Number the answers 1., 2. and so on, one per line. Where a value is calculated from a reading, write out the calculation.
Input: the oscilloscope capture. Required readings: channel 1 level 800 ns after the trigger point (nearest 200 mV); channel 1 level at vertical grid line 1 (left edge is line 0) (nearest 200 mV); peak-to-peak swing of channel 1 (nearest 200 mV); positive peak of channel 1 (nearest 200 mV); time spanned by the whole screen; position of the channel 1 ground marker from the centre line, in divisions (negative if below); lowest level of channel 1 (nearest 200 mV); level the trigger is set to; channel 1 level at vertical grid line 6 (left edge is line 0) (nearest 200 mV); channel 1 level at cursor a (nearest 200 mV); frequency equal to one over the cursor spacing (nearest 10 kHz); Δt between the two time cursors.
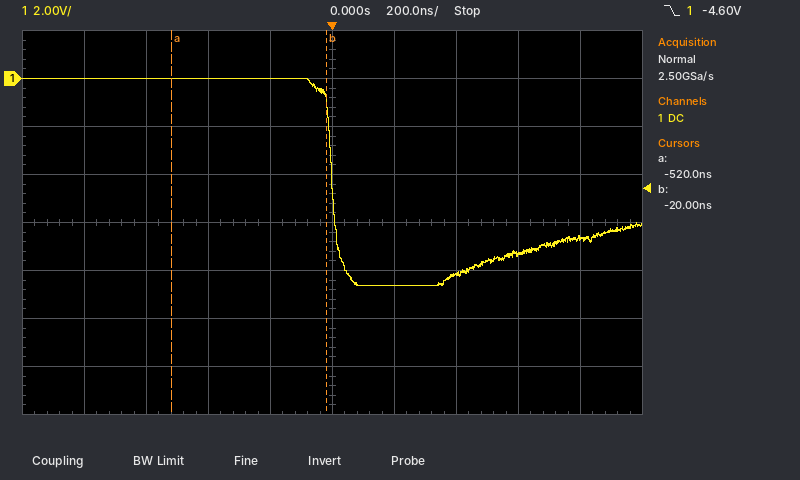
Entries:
1. -6.6 V
2. 0.0 V
3. 0.0 V − (-8.6 V) = 8.6 V
4. 0.0 V
5. 2 µs
6. +3.0 div
7. -8.6 V
8. -4.60 V
9. -8.6 V
10. 0.0 V
11. 1 / 500 ns ≈ 2.00 MHz
12. -20 ns − (-520 ns) = 500 ns
